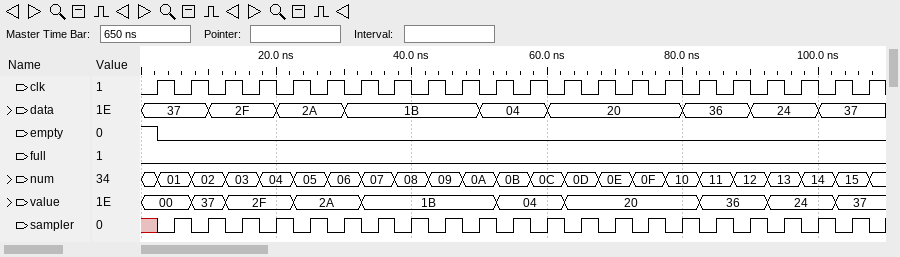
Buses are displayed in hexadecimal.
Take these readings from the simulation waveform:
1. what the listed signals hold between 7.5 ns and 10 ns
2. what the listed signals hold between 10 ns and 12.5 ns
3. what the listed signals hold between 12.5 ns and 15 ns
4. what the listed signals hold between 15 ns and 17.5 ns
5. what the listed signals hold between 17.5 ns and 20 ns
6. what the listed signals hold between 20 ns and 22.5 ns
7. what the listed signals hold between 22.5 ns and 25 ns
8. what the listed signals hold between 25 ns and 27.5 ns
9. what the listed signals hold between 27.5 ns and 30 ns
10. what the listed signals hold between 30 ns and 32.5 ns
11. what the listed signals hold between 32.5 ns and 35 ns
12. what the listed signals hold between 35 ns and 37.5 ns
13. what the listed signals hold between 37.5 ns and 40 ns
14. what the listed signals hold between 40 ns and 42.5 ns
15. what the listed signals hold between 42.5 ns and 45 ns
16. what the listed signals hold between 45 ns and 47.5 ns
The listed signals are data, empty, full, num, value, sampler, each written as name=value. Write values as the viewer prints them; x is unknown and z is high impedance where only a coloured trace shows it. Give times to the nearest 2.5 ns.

data=37, empty=0, full=0, num=02, value=37, sampler=0
data=2F, empty=0, full=0, num=02, value=37, sampler=1
data=2F, empty=0, full=0, num=03, value=2F, sampler=0
data=2F, empty=0, full=0, num=03, value=2F, sampler=1
data=2F, empty=0, full=0, num=04, value=2F, sampler=0
data=2A, empty=0, full=0, num=04, value=2F, sampler=1
data=2A, empty=0, full=0, num=05, value=2A, sampler=0
data=2A, empty=0, full=0, num=05, value=2A, sampler=1
data=2A, empty=0, full=0, num=06, value=2A, sampler=0
data=1B, empty=0, full=0, num=06, value=2A, sampler=1
data=1B, empty=0, full=0, num=07, value=1B, sampler=0
data=1B, empty=0, full=0, num=07, value=1B, sampler=1
data=1B, empty=0, full=0, num=08, value=1B, sampler=0
data=1B, empty=0, full=0, num=08, value=1B, sampler=1
data=1B, empty=0, full=0, num=09, value=1B, sampler=0
data=1B, empty=0, full=0, num=09, value=1B, sampler=1
